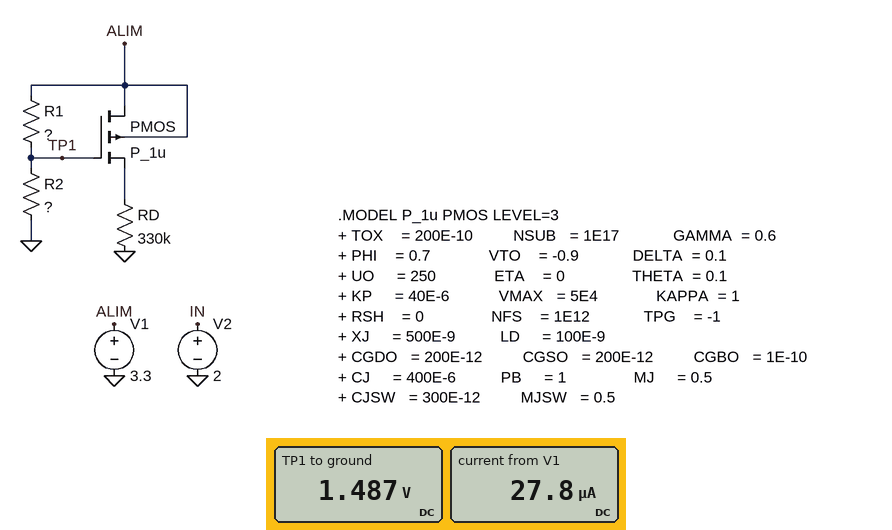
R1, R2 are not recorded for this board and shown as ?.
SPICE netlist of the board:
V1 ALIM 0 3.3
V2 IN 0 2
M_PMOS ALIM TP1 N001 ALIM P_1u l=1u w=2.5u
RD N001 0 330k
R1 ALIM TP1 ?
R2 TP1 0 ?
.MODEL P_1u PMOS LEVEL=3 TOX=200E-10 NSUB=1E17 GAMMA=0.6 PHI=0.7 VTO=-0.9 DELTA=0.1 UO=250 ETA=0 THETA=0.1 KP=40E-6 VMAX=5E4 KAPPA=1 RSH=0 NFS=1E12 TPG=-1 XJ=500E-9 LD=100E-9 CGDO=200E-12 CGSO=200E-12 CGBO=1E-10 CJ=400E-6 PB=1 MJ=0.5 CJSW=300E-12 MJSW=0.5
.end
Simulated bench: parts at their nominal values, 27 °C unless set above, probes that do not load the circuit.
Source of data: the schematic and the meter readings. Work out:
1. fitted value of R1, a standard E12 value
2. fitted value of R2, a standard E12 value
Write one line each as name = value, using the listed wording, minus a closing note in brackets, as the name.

fitted value of R1, a standard E12 value = 100 kΩ
fitted value of R2, a standard E12 value = 82 kΩ
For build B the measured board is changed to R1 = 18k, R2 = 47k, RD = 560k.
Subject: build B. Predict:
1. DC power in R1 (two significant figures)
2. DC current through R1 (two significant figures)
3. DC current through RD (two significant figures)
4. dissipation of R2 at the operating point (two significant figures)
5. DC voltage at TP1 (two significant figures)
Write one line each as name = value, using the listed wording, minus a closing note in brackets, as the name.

DC power in R1 = 46 µW
DC current through R1 = 51 µA
DC current through RD = 330 nA
dissipation of R2 at the operating point = 120 µW
DC voltage at TP1 = 2.4 V
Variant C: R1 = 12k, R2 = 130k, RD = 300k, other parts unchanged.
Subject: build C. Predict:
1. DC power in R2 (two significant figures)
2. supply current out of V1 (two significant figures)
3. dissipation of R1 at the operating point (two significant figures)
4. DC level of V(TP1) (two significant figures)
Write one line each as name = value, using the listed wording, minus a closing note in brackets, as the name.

DC power in R2 = 70 µW
supply current out of V1 = 23 µA
dissipation of R1 at the operating point = 6.5 µW
DC level of V(TP1) = 3.0 V
